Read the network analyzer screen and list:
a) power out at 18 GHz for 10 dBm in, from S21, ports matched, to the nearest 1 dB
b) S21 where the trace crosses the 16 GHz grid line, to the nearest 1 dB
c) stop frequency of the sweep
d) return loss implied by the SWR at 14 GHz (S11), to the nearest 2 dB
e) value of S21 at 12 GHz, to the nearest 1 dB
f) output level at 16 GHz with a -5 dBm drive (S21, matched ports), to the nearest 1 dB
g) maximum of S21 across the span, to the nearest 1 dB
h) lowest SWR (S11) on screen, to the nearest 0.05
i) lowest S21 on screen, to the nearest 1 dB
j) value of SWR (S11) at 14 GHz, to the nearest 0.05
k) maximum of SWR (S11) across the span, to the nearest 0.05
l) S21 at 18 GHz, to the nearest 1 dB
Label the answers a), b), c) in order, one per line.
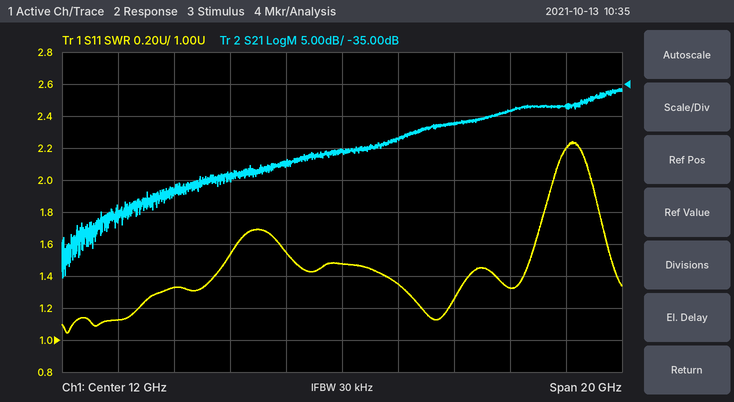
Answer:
a) -29 dBm
b) -41 dB
c) 22 GHz
d) 16 dB
e) -45 dB
f) -46 dBm
g) -36 dB
h) 1.05
i) -65 dB
j) 1.35
k) 2.25
l) -39 dB
